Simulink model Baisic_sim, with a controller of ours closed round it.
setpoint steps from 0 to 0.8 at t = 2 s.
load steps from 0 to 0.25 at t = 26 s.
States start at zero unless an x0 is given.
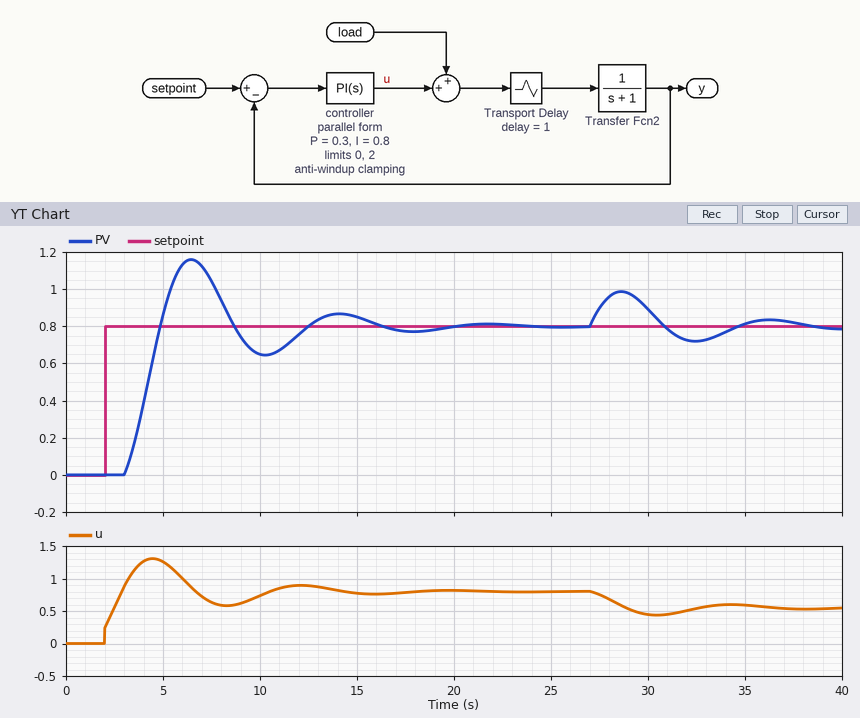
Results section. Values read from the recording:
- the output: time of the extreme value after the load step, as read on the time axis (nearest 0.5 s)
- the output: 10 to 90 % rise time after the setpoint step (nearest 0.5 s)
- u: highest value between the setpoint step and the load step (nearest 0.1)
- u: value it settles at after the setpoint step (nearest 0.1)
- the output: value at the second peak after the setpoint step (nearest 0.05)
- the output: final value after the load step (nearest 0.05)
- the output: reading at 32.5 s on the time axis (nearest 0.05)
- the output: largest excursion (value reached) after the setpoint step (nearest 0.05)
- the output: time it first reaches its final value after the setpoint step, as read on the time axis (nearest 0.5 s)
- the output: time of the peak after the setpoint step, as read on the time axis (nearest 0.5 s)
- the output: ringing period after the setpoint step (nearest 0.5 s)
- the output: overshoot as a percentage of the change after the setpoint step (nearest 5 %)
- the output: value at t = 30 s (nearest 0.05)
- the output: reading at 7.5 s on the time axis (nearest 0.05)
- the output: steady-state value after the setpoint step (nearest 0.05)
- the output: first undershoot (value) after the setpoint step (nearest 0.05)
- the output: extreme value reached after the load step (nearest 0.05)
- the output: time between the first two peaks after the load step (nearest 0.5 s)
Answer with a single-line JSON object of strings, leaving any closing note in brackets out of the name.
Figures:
{"the output: time of the extreme value after the load step, as read on the time axis": "28.5 s", "the output: 10 to 90 % rise time after the setpoint step": "1.5 s", "u: highest value between the setpoint step and the load step": "1.3", "u: value it settles at after the setpoint step": "0.8", "the output: value at the second peak after the setpoint step": "0.85", "the output: final value after the load step": "0.80", "the output: reading at 32.5 s on the time axis": "0.70", "the output: largest excursion (value reached) after the setpoint step": "1.15", "the output: time it first reaches its final value after the setpoint step, as read on the time axis": "5.0 s", "the output: time of the peak after the setpoint step, as read on the time axis": "6.5 s", "the output: ringing period after the setpoint step": "7.5 s", "the output: overshoot as a percentage of the change after the setpoint step": "45 %", "the output: value at t = 30 s": "0.90", "the output: reading at 7.5 s on the time axis": "1.05", "the output: steady-state value after the setpoint step": "0.80", "the output: first undershoot (value) after the setpoint step": "0.65", "the output: extreme value reached after the load step": "1.00", "the output: time between the first two peaks after the load step": "7.5 s"}
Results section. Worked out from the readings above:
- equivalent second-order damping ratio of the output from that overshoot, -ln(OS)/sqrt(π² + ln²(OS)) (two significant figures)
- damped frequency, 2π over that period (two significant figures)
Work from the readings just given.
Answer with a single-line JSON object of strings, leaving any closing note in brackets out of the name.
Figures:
{"equivalent second-order damping ratio of the output from that overshoot, -ln(OS)/sqrt(π² + ln²(OS))": "0.25", "damped frequency, 2π over that period": "0.84 rad/s"}
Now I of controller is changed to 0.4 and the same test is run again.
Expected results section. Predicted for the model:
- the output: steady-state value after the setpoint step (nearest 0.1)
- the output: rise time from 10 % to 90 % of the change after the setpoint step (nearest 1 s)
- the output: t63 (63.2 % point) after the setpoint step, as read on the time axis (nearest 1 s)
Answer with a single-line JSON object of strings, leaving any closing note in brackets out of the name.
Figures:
{"the output: steady-state value after the setpoint step": "0.8", "the output: rise time from 10 % to 90 % of the change after the setpoint step": "3 s", "the output: t63 (63.2 % point) after the setpoint step, as read on the time axis": "5 s"}
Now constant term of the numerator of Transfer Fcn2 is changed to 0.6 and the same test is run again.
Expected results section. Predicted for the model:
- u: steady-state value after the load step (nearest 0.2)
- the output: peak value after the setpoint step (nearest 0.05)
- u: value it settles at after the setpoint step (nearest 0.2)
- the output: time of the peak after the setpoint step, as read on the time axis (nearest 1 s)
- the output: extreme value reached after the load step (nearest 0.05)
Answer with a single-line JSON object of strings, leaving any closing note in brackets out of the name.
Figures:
{"u: steady-state value after the load step": "1.0", "the output: peak value after the setpoint step": "0.95", "u: value it settles at after the setpoint step": "1.4", "the output: time of the peak after the setpoint step, as read on the time axis": "8 s", "the output: extreme value reached after the load step": "0.90"}
